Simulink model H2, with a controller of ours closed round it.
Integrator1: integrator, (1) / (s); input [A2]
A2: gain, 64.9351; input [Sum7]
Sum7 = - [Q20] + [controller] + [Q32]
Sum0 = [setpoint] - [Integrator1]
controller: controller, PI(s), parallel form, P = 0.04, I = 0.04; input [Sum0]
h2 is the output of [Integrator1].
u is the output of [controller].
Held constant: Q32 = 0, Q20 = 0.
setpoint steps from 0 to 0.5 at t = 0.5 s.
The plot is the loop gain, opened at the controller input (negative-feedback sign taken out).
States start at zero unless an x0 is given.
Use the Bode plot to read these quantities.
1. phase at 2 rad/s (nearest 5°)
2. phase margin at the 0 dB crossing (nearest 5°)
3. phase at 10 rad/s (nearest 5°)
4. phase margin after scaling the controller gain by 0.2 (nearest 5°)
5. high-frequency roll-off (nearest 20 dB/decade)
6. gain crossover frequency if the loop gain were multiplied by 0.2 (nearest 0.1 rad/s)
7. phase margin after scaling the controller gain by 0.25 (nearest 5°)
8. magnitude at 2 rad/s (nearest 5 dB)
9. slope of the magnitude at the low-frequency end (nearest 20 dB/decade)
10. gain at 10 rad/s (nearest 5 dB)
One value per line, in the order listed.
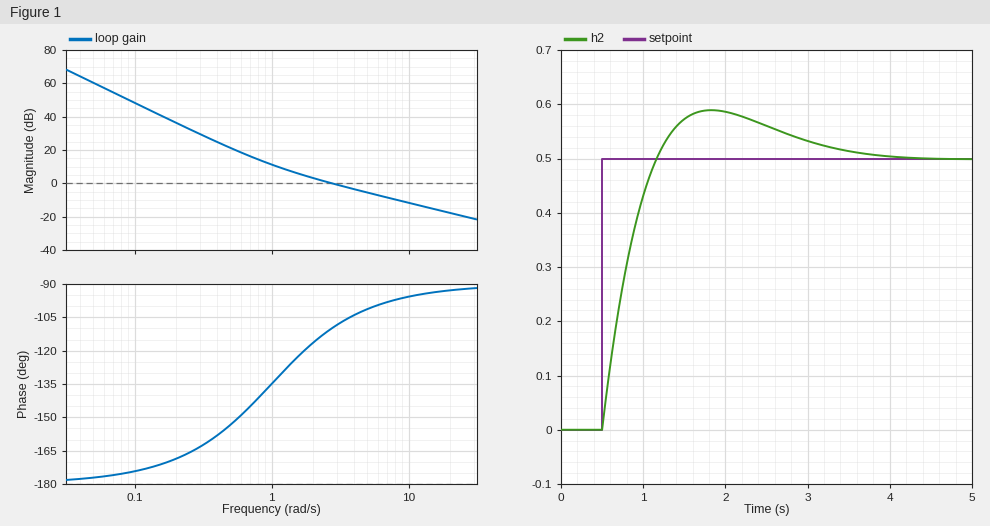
-115°
70°
-95°
40°
-20 dB/decade
0.8 rad/s
45°
5 dB
-40 dB/decade
-10 dB
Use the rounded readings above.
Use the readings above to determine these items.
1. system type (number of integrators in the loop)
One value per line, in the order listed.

2
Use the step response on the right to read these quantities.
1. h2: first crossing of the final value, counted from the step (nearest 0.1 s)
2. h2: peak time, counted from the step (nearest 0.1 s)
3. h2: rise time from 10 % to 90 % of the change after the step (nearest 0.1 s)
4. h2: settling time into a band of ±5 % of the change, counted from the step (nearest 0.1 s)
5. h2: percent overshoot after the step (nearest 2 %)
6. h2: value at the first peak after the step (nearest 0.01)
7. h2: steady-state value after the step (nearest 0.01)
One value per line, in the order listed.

0.7 s
1.3 s
0.5 s
2.7 s
18 %
0.59
0.50
